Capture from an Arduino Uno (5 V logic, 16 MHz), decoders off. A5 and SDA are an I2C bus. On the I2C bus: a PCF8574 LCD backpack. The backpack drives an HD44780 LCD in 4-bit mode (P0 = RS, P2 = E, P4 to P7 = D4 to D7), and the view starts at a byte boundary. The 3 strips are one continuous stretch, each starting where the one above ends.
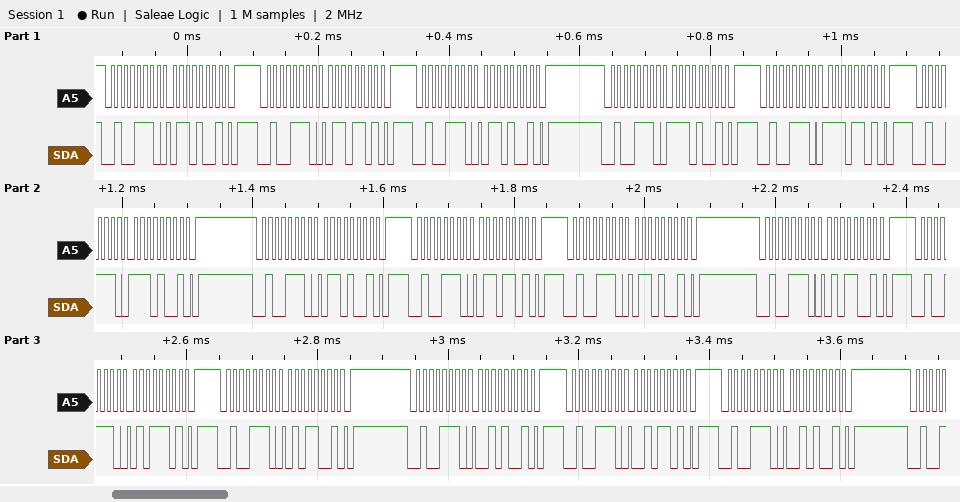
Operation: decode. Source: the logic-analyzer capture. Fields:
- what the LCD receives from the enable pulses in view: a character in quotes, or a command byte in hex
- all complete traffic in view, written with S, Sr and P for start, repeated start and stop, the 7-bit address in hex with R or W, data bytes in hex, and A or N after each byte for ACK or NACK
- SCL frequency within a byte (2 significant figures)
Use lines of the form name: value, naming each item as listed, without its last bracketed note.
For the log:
what the LCD receives from the enable pulses in view: a character in quotes, or a command byte in hex: 'n' 'e'
all complete traffic in view, written with S, Sr and P for start, repeated start and stop, the 7-bit address in hex with R or W, data bytes in hex, and A or N after each byte for ACK or NACK: S 27W A 69 A P S 27W A 6D A P S 27W A 69 A P S 27W A E9 A P S 27W A ED A P S 27W A E9 A P S 27W A 69 A P S 27W A 6D A P S 27W A 69 A P S 27W A 59 A P S 27W A 5D A P S 27W A 59 A P S 27W A 29 A P S 27W A 2D A P S 27W A 29 A P
SCL frequency within a byte: 100 kHz
